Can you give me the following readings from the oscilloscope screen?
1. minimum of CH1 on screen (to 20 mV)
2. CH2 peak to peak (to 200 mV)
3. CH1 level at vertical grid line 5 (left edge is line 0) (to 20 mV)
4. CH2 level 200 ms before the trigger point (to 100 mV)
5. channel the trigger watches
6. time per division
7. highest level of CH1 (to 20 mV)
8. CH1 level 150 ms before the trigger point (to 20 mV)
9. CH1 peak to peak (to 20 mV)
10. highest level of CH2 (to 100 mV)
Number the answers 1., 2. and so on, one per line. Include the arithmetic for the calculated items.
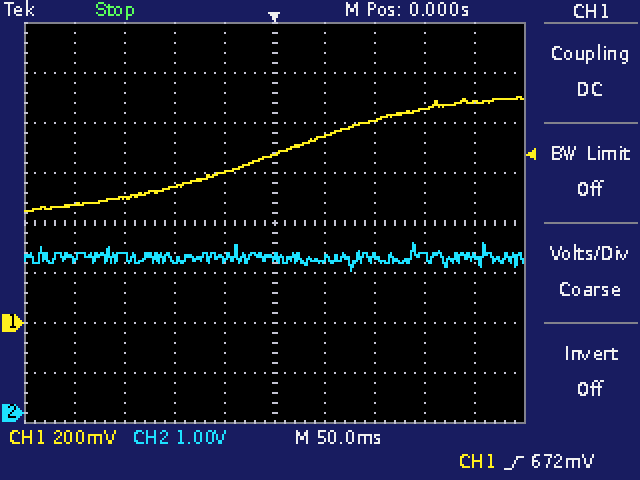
1. 440 mV
2. 600 mV
3. 680 mV
4. 3.1 V
5. CH1
6. 50 ms
7. 900 mV
8. 500 mV
9. 900 mV − (440 mV) = 460 mV
10. 3.4 V
